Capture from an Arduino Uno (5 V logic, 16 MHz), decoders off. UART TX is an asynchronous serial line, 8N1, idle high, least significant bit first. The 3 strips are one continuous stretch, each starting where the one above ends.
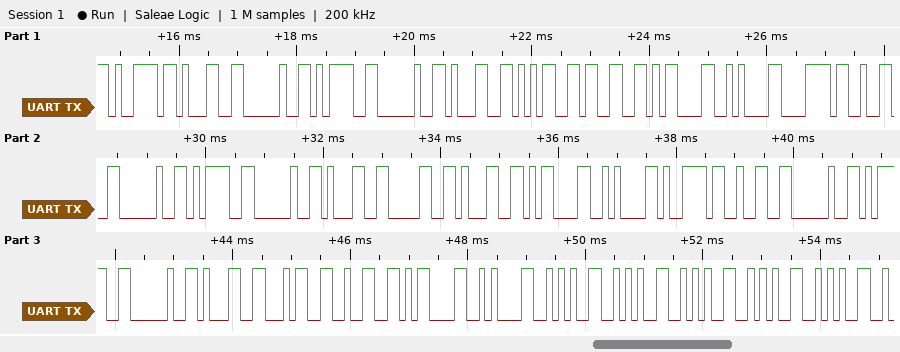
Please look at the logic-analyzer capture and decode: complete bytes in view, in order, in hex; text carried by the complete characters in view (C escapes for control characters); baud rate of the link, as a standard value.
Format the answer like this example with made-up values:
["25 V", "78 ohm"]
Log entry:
["79 31 20 3D 20 31 35 33 0D 0A 78 32 20 3D 20 31 30 31 0D 0A 79 32 20 3D 20 31 34 32 0D 0A 2A 2A 2A 2A 2A", "\"y1 = 153\\r\\nx2 = 101\\r\\ny2 = 142\\r\\n*****\"", "9600 baud"]
